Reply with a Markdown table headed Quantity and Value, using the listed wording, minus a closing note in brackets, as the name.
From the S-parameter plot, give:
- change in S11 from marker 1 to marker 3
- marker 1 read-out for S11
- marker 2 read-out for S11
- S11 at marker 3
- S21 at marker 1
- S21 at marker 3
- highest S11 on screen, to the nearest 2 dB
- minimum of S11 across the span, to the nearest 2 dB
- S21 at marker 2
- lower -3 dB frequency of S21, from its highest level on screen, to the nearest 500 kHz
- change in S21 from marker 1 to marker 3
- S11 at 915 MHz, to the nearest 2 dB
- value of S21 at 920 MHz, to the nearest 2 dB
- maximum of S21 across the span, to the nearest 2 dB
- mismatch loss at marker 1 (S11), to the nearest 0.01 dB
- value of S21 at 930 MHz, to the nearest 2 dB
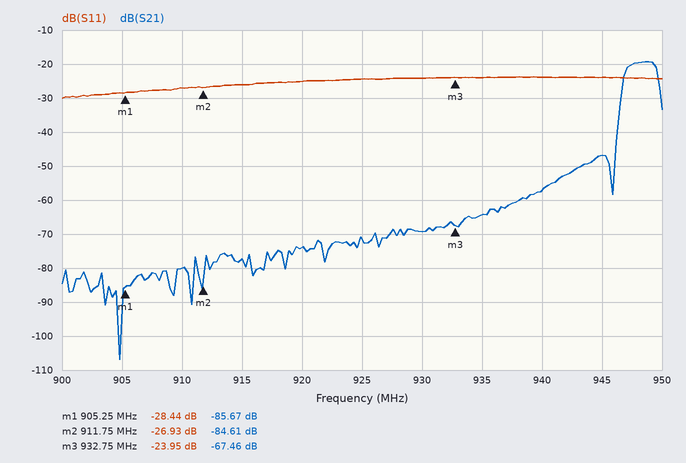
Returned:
| Quantity | Value |
|---|---|
| change in S11 from marker 1 to marker 3 | 4.49 dB |
| marker 1 read-out for S11 | -28.44 dB |
| marker 2 read-out for S11 | -26.93 dB |
| S11 at marker 3 | -23.95 dB |
| S21 at marker 1 | -85.67 dB |
| S21 at marker 3 | -67.46 dB |
| highest S11 on screen, to the nearest 2 dB | -24 dB |
| minimum of S11 across the span, to the nearest 2 dB | -30 dB |
| S21 at marker 2 | -84.61 dB |
| lower -3 dB frequency of S21, from its highest level on screen, to the nearest 500 kHz | 947.0 MHz |
| change in S21 from marker 1 to marker 3 | 18.21 dB |
| S11 at 915 MHz, to the nearest 2 dB | -26 dB |
| value of S21 at 920 MHz, to the nearest 2 dB | -74 dB |
| maximum of S21 across the span, to the nearest 2 dB | -20 dB |
| mismatch loss at marker 1 (S11), to the nearest 0.01 dB | 0.01 dB |
| value of S21 at 930 MHz, to the nearest 2 dB | -70 dB |
